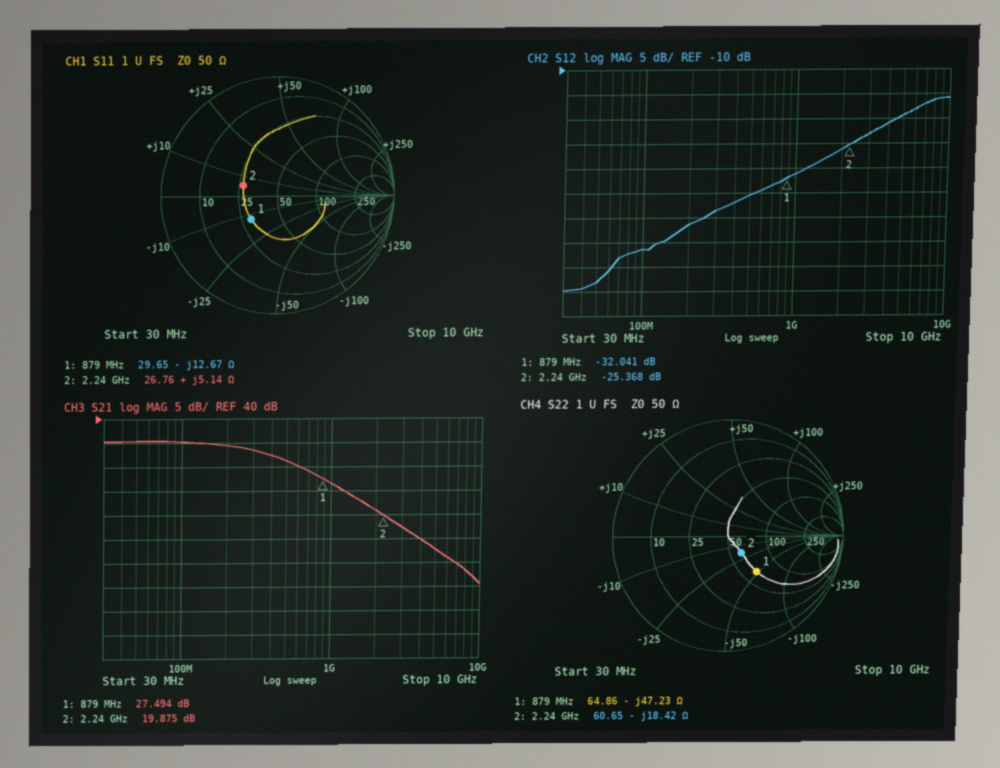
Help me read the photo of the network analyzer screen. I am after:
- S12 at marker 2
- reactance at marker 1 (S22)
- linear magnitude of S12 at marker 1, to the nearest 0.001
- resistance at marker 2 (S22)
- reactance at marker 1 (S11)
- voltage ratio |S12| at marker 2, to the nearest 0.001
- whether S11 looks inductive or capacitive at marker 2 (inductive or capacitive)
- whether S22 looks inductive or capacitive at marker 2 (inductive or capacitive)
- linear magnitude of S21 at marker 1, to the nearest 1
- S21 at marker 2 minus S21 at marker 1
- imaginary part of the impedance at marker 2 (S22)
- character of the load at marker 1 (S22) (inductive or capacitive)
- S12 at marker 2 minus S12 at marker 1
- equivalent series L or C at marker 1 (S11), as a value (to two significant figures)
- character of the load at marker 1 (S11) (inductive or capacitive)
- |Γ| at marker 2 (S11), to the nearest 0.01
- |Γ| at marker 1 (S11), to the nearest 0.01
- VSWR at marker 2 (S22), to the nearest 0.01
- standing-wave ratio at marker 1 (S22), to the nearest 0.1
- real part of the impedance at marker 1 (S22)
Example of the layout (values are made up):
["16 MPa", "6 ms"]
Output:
["-25.368 dB", "-47.23 Ω", "0.025", "60.65 Ω", "-12.67 Ω", "0.054", "inductive", "capacitive", "24", "-7.619 dB", "-18.42 Ω", "capacitive", "6.673 dB", "14 pF", "capacitive", "0.31", "0.30", "1.47", "2.3", "64.86 Ω"]
